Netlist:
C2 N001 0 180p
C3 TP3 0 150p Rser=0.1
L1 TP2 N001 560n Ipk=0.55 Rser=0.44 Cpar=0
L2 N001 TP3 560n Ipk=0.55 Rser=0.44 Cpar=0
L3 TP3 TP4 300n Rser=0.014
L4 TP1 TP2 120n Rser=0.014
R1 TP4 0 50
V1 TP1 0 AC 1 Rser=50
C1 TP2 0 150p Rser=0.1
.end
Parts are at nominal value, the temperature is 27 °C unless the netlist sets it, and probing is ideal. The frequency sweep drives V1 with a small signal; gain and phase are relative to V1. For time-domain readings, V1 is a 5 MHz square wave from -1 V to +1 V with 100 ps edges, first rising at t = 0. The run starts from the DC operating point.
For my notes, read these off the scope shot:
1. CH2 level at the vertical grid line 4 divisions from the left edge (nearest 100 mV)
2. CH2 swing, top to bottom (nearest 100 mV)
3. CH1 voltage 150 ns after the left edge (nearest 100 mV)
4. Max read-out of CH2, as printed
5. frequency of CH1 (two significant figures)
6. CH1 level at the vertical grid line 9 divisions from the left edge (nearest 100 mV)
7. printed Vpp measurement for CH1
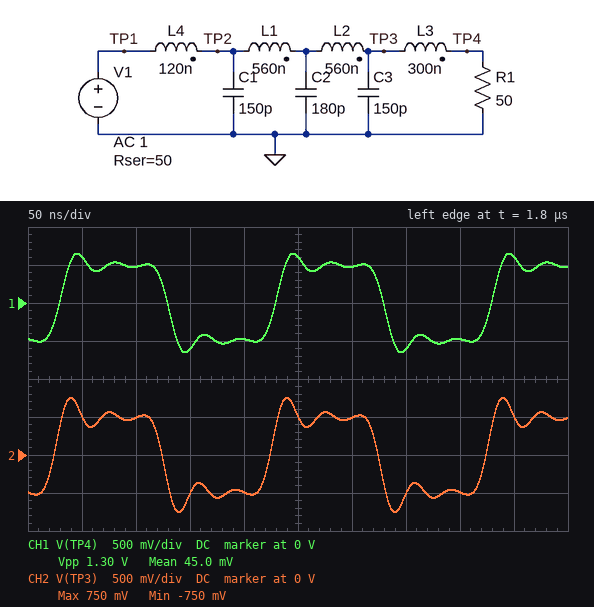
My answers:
-500 mV
1.5 V
-600 mV
750 mV
5.0 MHz
600 mV
1.30 V
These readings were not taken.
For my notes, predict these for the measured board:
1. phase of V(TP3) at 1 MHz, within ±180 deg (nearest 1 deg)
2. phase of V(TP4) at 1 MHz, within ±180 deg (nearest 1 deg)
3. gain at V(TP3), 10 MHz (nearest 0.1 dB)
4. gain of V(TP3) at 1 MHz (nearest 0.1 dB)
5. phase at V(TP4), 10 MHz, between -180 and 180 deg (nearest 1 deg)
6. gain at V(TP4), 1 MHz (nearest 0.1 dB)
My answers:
-8 deg
-10 deg
-5.6 dB
-6.1 dB
-99 deg
-6.1 dB
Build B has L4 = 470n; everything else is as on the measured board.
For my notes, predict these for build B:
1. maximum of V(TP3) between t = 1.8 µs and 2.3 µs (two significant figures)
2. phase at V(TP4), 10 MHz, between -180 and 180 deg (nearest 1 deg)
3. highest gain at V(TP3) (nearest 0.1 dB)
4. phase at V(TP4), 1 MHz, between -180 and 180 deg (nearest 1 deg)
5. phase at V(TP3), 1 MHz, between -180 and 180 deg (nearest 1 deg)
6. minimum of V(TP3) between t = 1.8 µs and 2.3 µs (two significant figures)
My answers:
740 mV
-111 deg
-3.0 dB
-11 deg
-9 deg
-740 mV
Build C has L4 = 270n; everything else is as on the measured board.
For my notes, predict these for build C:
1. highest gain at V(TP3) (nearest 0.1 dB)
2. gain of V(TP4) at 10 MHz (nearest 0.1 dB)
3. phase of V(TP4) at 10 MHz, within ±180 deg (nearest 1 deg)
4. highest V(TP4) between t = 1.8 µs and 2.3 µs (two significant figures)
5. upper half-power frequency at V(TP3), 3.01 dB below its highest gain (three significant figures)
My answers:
-3.1 dB
-6.1 dB
-104 deg
660 mV
31.5 MHz
